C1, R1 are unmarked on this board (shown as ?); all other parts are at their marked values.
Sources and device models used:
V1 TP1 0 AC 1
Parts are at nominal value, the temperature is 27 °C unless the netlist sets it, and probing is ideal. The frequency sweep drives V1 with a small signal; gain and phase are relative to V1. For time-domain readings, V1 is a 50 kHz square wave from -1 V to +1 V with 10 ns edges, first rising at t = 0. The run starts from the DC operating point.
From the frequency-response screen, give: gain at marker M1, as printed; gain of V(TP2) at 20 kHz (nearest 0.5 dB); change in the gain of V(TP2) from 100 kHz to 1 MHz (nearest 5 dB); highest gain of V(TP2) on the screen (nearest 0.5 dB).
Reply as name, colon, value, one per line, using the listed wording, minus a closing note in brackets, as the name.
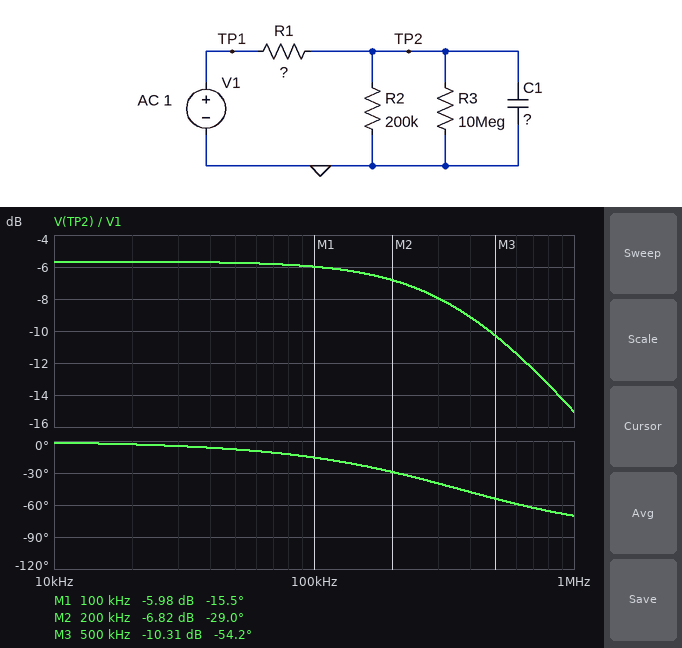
gain at marker M1, as printed: -5.98 dB
gain of V(TP2) at 20 kHz: -5.5 dB
change in the gain of V(TP2) from 100 kHz to 1 MHz: -10 dB
highest gain of V(TP2) on the screen: -5.5 dB
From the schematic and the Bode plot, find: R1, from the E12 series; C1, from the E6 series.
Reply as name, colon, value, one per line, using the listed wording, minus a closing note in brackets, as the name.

R1, from the E12 series: 180 kΩ
C1, from the E6 series: 4.7 pF
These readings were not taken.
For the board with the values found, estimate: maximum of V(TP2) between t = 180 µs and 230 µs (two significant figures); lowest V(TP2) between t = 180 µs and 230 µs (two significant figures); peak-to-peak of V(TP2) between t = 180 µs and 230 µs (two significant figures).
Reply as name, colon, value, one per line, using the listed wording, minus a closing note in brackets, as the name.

maximum of V(TP2) between t = 180 µs and 230 µs: 520 mV
lowest V(TP2) between t = 180 µs and 230 µs: -520 mV
peak-to-peak of V(TP2) between t = 180 µs and 230 µs: 1.0 V
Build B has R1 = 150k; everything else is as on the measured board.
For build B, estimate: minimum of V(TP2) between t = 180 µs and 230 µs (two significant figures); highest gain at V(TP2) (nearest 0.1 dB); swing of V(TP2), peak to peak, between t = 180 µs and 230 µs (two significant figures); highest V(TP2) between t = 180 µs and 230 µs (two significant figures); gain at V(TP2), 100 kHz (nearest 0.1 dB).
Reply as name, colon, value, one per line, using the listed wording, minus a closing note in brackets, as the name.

minimum of V(TP2) between t = 180 µs and 230 µs: -570 mV
highest gain at V(TP2): -4.9 dB
swing of V(TP2), peak to peak, between t = 180 µs and 230 µs: 1.1 V
highest V(TP2) between t = 180 µs and 230 µs: 570 mV
gain at V(TP2), 100 kHz: -5.2 dB
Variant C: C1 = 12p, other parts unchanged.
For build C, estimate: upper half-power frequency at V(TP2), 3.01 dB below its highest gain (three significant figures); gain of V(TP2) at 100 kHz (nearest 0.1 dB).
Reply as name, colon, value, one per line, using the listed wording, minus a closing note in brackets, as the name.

upper half-power frequency at V(TP2), 3.01 dB below its highest gain: 141 kHz
gain of V(TP2) at 100 kHz: -7.4 dB
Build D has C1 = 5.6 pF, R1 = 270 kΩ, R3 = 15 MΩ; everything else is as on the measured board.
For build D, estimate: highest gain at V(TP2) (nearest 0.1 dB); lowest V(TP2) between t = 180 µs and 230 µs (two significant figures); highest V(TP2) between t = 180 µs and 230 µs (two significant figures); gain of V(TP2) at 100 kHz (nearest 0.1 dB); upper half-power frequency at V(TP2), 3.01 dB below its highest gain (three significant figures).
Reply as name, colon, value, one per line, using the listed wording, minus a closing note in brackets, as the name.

highest gain at V(TP2): -7.5 dB
lowest V(TP2) between t = 180 µs and 230 µs: -420 mV
highest V(TP2) between t = 180 µs and 230 µs: 420 mV
gain of V(TP2) at 100 kHz: -8.1 dB
upper half-power frequency at V(TP2), 3.01 dB below its highest gain: 249 kHz
